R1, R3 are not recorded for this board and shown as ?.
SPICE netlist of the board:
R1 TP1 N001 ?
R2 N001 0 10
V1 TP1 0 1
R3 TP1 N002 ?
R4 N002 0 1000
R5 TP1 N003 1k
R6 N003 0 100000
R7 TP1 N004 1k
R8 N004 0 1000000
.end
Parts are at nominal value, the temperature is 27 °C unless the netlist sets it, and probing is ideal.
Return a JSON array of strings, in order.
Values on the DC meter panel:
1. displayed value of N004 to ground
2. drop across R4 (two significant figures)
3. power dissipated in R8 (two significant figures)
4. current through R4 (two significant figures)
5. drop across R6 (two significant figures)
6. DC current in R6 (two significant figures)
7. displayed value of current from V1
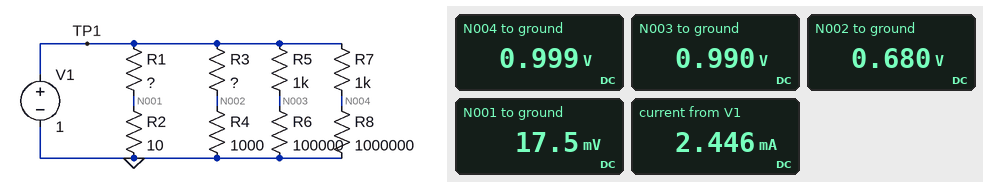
["0.999 V", "680 mV", "1.0 µW", "680 µA", "990 mV", "9.9 µA", "2.446 mA"]
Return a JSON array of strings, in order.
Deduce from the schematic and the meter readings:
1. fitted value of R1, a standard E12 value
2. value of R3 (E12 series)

["560 Ω", "470 Ω"]
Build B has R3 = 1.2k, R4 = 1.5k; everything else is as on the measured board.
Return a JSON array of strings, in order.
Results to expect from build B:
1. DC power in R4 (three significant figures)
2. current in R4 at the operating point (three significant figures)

["206 µW", "370 µA"]
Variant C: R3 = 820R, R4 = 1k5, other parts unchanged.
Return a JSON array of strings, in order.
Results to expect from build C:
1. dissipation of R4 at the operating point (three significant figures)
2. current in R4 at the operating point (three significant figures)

["279 µW", "431 µA"]
